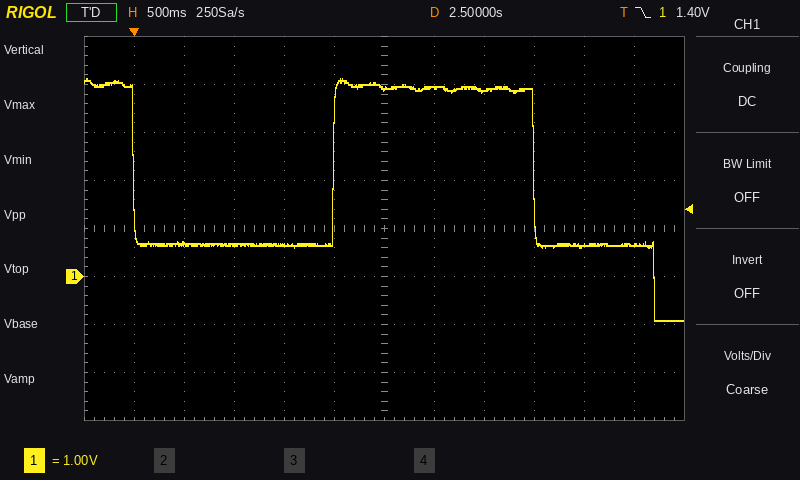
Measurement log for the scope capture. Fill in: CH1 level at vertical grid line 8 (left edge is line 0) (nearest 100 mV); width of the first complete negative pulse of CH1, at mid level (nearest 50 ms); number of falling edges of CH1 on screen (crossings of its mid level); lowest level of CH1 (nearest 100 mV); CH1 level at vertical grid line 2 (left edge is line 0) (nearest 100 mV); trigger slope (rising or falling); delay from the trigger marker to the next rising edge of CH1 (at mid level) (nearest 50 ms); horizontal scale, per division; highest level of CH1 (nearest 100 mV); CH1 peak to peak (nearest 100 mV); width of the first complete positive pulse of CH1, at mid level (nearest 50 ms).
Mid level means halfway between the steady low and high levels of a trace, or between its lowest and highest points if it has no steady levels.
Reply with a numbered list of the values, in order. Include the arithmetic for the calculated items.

1. 3.9 V
2. 2.00 s
3. 2
4. -900 mV
5. 700 mV
6. falling
7. 2.00 s
8. 500 ms
9. 4.1 V
10. 4.1 V − (-900 mV) = 5.0 V
11. 2.00 s
